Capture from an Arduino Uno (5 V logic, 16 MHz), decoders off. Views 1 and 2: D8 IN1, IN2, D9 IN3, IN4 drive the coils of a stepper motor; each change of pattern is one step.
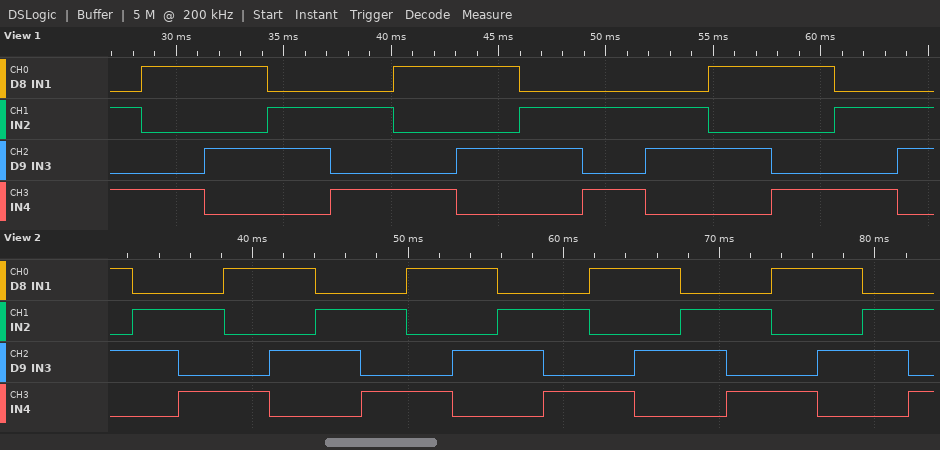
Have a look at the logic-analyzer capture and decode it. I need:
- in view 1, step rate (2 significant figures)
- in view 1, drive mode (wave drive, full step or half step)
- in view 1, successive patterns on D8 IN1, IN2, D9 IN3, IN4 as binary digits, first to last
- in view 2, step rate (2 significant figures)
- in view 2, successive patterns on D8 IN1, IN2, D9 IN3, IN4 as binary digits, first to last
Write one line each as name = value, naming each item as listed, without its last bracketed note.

in view 1, step rate = 340 steps/s
in view 1, drive mode = full step
in view 1, successive patterns on D8 IN1, IN2, D9 IN3, IN4 as binary digits, first to last = 0101 1001 1010 0110 0101 1001 1010 0110 0101 0110 1010 1001 0101 0110
in view 2, step rate = 340 steps/s
in view 2, successive patterns on D8 IN1, IN2, D9 IN3, IN4 as binary digits, first to last = 1010 0110 0101 1001 1010 0110 0101 1001 1010 0110 0101 1001 1010 0110 0101 1001 1010 0110 0101
